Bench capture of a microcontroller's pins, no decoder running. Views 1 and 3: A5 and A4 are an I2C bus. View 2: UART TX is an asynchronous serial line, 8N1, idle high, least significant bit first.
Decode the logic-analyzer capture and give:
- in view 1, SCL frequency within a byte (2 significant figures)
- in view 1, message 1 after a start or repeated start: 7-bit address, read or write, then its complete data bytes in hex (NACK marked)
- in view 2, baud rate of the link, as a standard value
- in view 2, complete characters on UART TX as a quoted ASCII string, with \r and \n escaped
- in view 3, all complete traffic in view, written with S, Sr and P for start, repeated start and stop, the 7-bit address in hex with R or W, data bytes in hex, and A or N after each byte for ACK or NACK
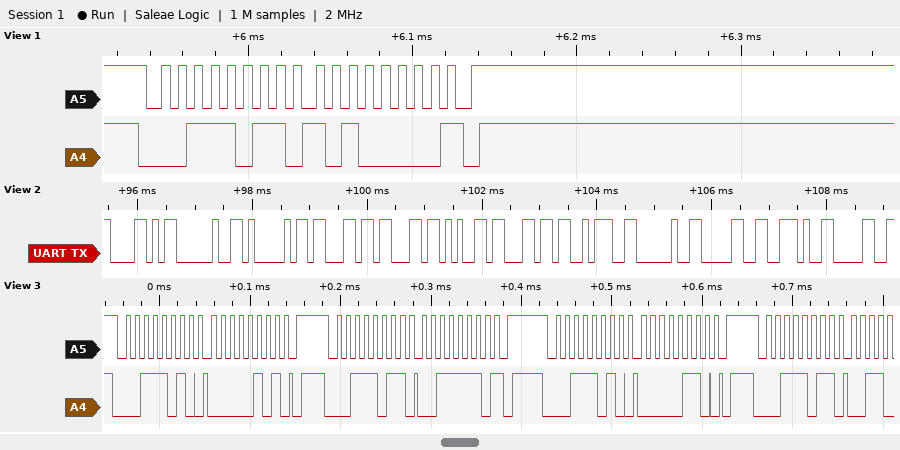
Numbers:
100 kHz
0x1D read: A0 NACK
9600 baud
"X Accel: 0.0"
S 1DW A 05 A P S 1DR A 3E N P S 1DW A 06 A P S 1DR A
